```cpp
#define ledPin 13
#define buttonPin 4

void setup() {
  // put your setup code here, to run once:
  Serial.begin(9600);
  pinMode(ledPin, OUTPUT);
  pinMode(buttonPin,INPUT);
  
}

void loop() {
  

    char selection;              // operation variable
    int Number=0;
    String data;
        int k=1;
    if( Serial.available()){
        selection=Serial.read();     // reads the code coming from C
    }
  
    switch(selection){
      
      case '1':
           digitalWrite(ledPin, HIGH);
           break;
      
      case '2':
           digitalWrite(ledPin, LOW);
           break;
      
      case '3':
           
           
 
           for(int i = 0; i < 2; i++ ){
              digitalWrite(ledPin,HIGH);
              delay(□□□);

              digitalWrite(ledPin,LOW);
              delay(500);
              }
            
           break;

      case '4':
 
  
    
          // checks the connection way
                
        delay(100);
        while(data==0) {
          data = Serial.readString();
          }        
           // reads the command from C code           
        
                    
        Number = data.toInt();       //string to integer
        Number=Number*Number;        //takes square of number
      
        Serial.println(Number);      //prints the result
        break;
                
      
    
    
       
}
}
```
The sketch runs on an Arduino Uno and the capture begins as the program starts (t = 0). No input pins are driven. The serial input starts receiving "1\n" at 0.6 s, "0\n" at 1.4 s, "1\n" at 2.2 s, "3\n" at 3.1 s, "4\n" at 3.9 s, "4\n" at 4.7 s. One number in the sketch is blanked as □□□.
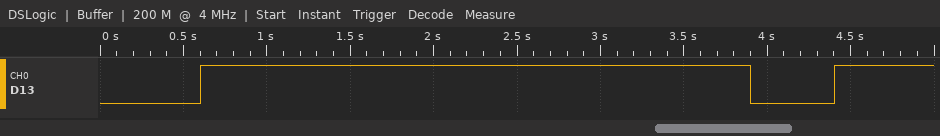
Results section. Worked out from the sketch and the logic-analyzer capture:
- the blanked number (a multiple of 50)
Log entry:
800
